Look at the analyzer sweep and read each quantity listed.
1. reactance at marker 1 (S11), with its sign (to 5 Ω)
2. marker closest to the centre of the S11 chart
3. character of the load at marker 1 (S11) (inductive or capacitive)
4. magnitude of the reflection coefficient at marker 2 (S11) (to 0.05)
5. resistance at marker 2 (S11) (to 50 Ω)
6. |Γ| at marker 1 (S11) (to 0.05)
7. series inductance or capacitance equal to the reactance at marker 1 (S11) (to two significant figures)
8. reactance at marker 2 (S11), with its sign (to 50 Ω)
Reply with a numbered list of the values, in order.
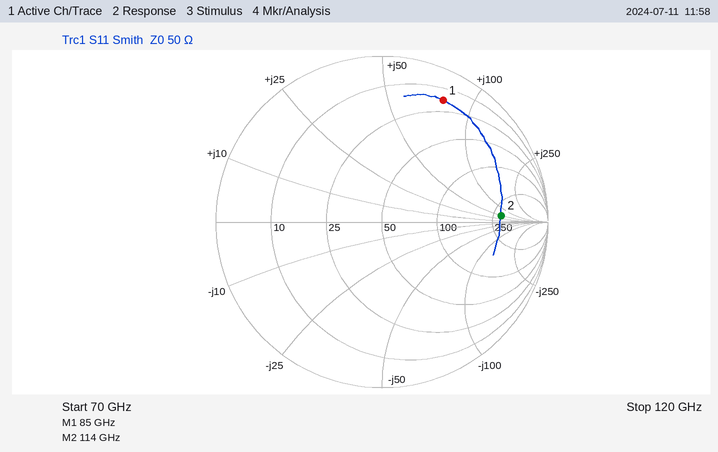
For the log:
1. +80 Ω
2. marker 2
3. inductive
4. 0.70
5. 300 Ω
6. 0.80
7. 150 pH
8. +50 Ω
